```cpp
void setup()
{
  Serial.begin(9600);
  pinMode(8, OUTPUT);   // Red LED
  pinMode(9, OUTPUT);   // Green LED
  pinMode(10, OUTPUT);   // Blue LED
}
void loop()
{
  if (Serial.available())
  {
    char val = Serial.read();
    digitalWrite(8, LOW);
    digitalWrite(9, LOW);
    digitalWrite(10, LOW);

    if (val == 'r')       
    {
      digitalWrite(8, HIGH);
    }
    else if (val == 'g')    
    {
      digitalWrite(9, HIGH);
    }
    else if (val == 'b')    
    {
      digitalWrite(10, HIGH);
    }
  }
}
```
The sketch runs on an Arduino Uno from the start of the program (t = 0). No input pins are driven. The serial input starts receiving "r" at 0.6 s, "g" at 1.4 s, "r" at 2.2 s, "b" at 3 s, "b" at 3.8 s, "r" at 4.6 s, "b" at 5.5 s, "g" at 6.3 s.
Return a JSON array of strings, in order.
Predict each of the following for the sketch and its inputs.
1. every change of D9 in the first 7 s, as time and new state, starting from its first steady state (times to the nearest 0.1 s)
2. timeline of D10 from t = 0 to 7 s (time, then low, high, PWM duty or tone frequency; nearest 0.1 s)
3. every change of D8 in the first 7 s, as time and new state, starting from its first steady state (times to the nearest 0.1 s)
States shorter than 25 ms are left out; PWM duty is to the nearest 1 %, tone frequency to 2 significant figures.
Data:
["0 s low; 1.4 s high; 2.2 s low; 6.3 s high", "0 s low; 3 s high; 4.6 s low; 5.5 s high; 6.3 s low", "0 s low; 0.6 s high; 1.4 s low; 2.2 s high; 3 s low; 4.6 s high; 5.5 s low"]
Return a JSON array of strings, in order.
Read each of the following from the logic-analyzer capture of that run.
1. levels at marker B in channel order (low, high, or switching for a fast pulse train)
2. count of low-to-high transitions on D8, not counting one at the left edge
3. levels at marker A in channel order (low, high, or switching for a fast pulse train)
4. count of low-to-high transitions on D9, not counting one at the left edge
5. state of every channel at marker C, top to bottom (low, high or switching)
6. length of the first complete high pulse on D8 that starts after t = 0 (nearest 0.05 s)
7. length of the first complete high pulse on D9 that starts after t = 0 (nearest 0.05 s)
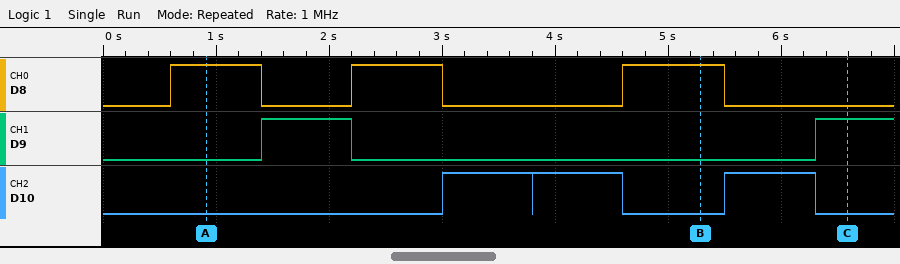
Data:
["D8 high, D9 low, D10 low", "3", "D8 high, D9 low, D10 low", "2", "D8 low, D9 high, D10 low", "0.80 s", "0.80 s"]
